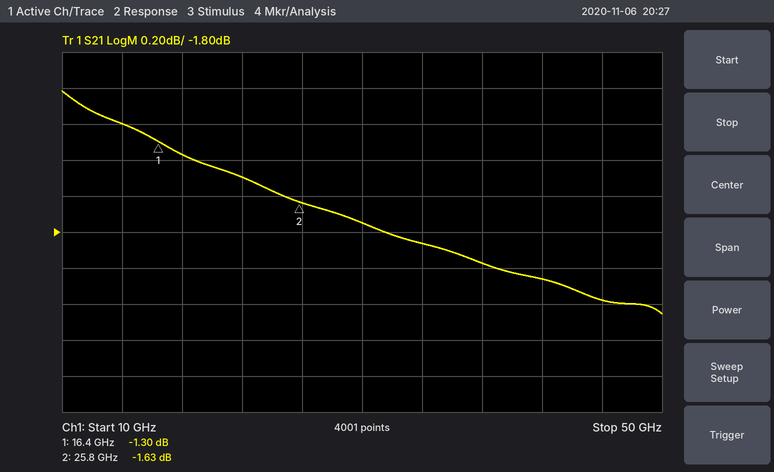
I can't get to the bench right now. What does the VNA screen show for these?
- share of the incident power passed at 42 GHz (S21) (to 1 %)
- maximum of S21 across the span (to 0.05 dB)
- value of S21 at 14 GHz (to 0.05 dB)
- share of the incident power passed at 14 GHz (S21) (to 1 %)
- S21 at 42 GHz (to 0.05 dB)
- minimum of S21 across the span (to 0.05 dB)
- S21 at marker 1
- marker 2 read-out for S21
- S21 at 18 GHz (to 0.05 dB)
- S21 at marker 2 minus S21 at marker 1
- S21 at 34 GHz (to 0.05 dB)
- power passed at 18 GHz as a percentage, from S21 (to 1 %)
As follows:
62 %
-1.00 dB
-1.20 dB
76 %
-2.05 dB
-2.25 dB
-1.30 dB
-1.63 dB
-1.35 dB
-0.33 dB
-1.85 dB
73 %
